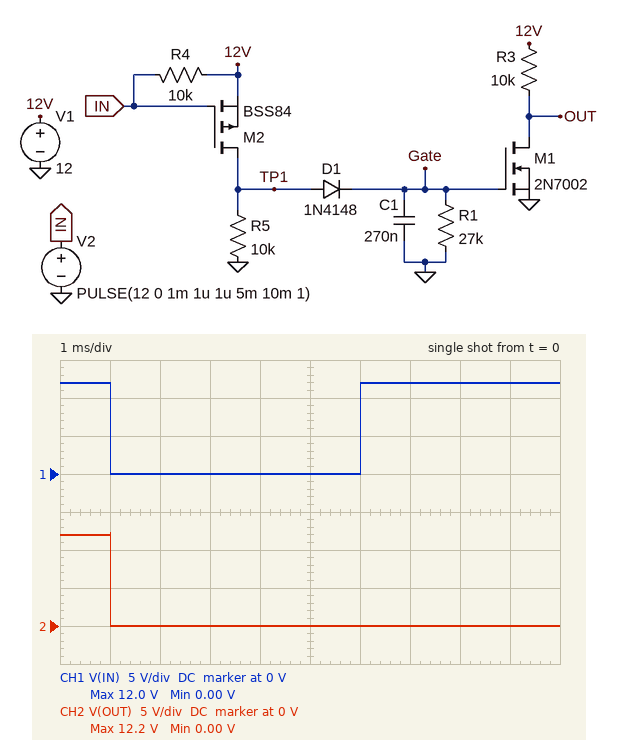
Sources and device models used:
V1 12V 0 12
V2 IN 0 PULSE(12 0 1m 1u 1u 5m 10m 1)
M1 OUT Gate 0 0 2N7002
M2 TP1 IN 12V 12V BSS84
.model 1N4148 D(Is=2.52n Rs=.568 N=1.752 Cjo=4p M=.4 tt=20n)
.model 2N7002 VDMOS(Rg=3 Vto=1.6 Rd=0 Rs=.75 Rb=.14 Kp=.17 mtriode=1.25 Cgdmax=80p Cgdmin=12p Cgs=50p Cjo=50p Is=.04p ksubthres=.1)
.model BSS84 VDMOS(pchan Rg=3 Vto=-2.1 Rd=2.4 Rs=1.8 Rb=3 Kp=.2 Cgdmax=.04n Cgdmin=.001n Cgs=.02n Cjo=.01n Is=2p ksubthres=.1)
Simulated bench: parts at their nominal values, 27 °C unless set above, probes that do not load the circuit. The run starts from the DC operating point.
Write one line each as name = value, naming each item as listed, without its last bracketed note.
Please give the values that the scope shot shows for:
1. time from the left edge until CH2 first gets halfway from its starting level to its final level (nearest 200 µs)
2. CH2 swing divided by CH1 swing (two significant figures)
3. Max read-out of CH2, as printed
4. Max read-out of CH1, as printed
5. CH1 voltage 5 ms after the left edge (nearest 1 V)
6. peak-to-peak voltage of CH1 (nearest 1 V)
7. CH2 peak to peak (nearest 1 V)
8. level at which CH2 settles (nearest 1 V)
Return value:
time from the left edge until CH2 first gets halfway from its starting level to its final level = 1.0 ms
CH2 swing divided by CH1 swing = 1.0
Max read-out of CH2, as printed = 12.2 V
Max read-out of CH1, as printed = 12.0 V
CH1 voltage 5 ms after the left edge = 0 V
peak-to-peak voltage of CH1 = 12 V
CH2 peak to peak = 12 V
level at which CH2 settles = 0 V
